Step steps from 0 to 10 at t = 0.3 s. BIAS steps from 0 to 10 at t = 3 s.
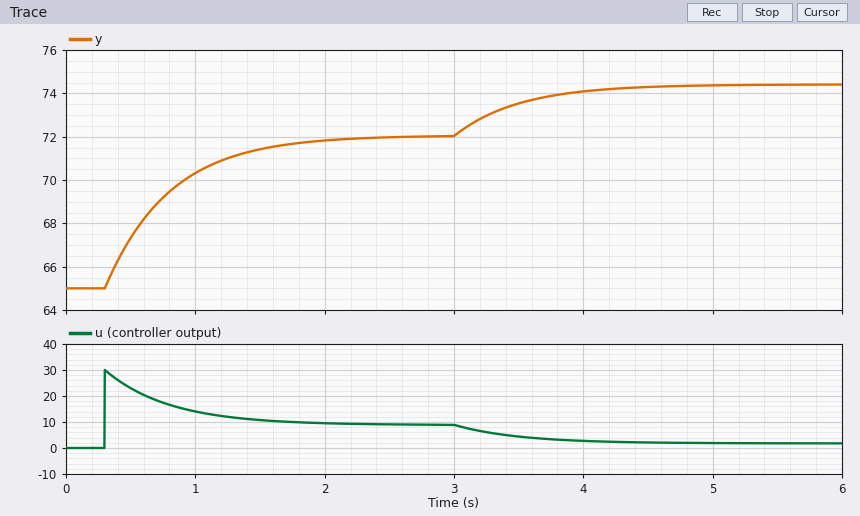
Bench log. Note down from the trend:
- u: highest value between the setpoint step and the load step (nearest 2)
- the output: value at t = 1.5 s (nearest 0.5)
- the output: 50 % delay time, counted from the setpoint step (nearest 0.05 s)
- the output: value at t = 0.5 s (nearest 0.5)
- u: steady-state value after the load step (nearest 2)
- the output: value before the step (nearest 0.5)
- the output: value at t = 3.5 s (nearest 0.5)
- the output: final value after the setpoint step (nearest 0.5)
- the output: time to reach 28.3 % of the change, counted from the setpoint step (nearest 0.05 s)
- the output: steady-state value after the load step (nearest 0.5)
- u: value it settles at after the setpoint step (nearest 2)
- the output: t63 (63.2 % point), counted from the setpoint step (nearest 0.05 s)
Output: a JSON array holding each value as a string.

["30", "71.5", "0.35 s", "67.5", "2", "65.0", "73.5", "72.0", "0.15 s", "74.5", "8", "0.50 s"]
